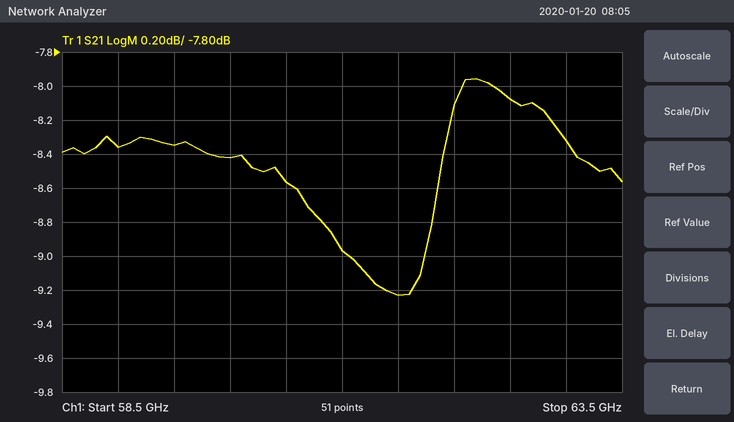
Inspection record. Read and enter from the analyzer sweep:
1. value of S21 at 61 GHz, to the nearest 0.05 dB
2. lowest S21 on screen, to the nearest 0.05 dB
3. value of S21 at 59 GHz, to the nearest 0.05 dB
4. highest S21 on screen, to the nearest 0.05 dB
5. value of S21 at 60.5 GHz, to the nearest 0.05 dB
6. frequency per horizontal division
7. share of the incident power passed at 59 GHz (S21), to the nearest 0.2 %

-8.95 dB
-9.25 dB
-8.35 dB
-7.95 dB
-8.55 dB
500 MHz
14.6 %
